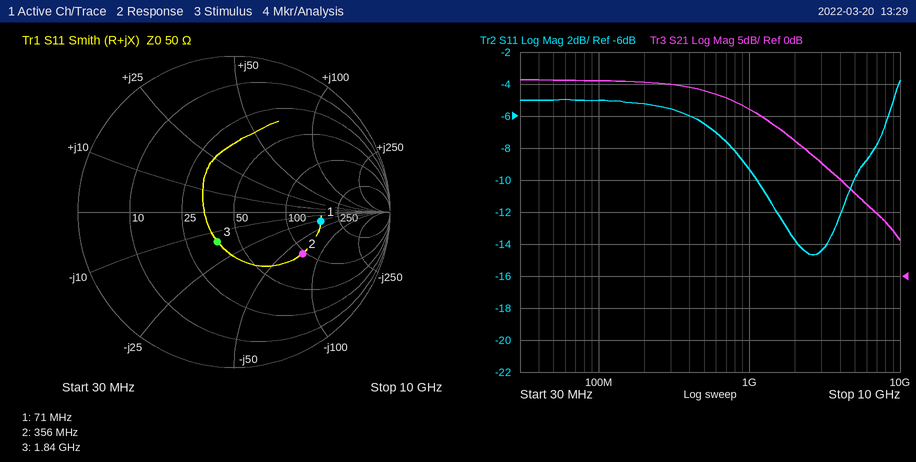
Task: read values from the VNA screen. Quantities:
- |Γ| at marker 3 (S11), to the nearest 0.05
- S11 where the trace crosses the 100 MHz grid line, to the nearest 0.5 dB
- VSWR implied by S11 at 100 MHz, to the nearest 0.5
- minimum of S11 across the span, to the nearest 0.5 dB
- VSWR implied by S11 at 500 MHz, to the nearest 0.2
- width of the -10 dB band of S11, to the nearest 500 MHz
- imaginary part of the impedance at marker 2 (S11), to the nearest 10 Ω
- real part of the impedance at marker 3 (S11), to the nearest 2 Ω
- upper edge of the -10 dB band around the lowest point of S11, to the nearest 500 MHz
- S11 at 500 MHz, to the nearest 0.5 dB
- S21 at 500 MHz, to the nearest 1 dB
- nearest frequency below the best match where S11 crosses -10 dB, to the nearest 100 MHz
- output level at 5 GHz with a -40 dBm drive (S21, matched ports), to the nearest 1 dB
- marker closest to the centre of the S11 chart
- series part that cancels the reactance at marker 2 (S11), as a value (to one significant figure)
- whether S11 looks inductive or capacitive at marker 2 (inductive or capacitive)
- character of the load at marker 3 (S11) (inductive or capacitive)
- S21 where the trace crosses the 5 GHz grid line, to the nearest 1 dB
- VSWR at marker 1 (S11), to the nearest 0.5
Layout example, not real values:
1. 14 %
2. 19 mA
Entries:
1. 0.20
2. -5.0 dB
3. 3.5
4. -14.5 dB
5. 2.8
6. 4.0 GHz
7. -70 Ω
8. 38 Ω
9. 5.0 GHz
10. -6.5 dB
11. 29 dB
12. 1.1 GHz
13. -27 dBm
14. marker 3
15. 30 nH
16. capacitive
17. capacitive
18. 13 dB
19. 3.5
